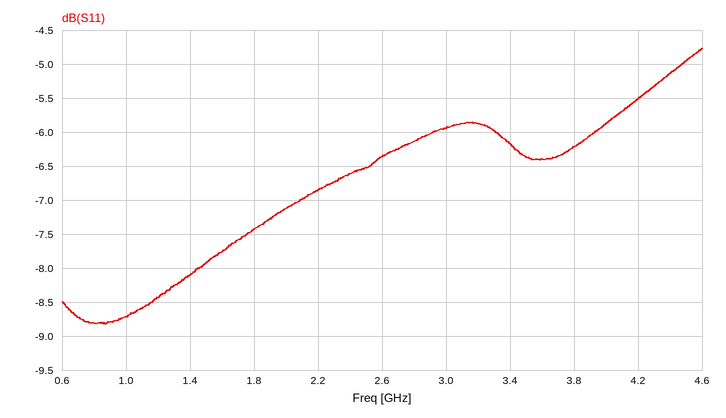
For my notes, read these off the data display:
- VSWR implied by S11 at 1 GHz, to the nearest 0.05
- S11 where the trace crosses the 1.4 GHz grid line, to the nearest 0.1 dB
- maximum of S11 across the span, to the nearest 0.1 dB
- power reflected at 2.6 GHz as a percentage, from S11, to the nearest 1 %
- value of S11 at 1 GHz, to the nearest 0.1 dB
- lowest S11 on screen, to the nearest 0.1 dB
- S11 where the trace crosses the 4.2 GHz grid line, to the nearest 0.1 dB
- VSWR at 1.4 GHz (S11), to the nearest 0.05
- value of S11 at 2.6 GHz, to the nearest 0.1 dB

2.15
-8.1 dB
-4.8 dB
23 %
-8.7 dB
-8.8 dB
-5.5 dB
2.30
-6.4 dB
